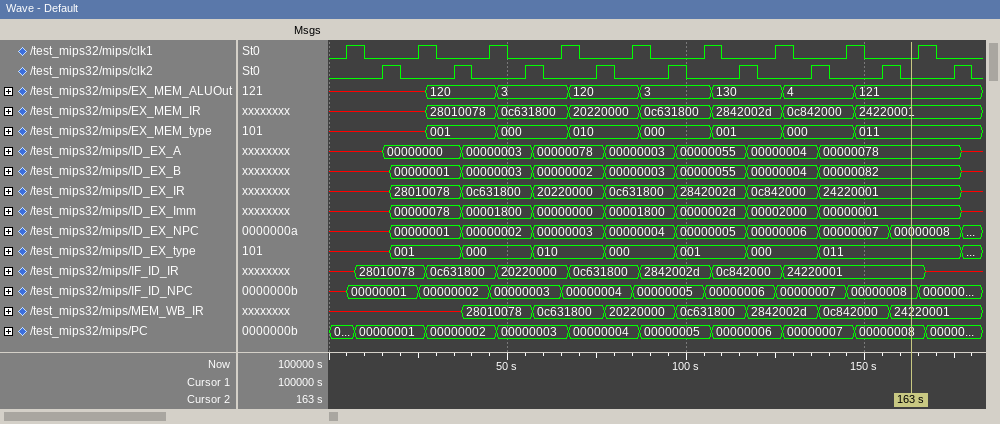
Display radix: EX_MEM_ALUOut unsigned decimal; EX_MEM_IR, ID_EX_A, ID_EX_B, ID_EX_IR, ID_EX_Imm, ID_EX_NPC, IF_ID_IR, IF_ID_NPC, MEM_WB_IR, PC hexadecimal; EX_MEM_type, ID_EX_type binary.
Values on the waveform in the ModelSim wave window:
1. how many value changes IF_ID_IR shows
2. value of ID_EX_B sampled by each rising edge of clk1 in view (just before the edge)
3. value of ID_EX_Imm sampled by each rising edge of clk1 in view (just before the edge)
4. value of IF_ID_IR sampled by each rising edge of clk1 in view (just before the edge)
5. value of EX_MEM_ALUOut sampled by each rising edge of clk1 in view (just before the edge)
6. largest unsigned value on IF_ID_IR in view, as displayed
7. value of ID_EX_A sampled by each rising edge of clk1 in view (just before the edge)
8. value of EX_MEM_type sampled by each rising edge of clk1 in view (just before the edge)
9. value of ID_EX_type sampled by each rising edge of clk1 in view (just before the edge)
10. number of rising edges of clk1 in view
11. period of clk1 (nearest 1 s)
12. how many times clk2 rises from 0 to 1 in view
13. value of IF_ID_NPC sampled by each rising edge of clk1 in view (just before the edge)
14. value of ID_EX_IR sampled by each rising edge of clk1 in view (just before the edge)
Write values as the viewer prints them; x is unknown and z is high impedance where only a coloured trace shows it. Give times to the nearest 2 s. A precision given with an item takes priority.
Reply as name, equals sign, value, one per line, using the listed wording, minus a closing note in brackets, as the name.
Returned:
how many value changes IF_ID_IR shows = 8
value of ID_EX_B sampled by each rising edge of clk1 in view = x, 00000001, 00000003, 00000002, 00000003, 00000055, 00000004, 00000082, 00000082
value of ID_EX_Imm sampled by each rising edge of clk1 in view = x, 00000078, 00001800, 00000000, 00001800, 0000002d, 00002000, 00000001, 00000001
value of IF_ID_IR sampled by each rising edge of clk1 in view = x, 28010078, 0c631800, 20220000, 0c631800, 2842002d, 0c842000, 24220001, 24220001
value of EX_MEM_ALUOut sampled by each rising edge of clk1 in view = x, x, 120, 3, 120, 3, 130, 4, 121
largest unsigned value on IF_ID_IR in view, as displayed = 2842002d
value of ID_EX_A sampled by each rising edge of clk1 in view = x, 00000000, 00000003, 00000078, 00000003, 00000055, 00000004, 00000078, 00000078
value of EX_MEM_type sampled by each rising edge of clk1 in view = x, x, 001, 000, 010, 000, 001, 000, 011
value of ID_EX_type sampled by each rising edge of clk1 in view = x, 001, 000, 010, 000, 001, 000, 011, 011
number of rising edges of clk1 in view = 9
period of clk1 = 20 s
how many times clk2 rises from 0 to 1 in view = 9
value of IF_ID_NPC sampled by each rising edge of clk1 in view = x, 00000001, 00000002, 00000003, 00000004, 00000005, 00000006, 00000007, 00000008
value of ID_EX_IR sampled by each rising edge of clk1 in view = x, 28010078, 0c631800, 20220000, 0c631800, 2842002d, 0c842000, 24220001, 24220001
